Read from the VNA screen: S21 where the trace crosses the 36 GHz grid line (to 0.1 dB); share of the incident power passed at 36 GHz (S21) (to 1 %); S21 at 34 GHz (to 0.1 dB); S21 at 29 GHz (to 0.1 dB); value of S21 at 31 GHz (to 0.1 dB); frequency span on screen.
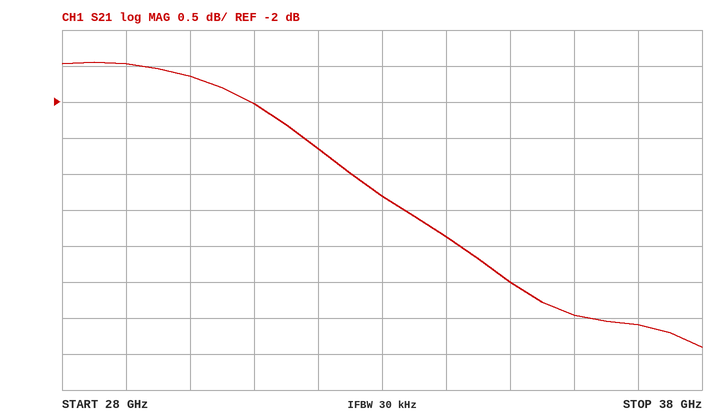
-5.0 dB
32 %
-3.9 dB
-1.5 dB
-2.0 dB
10 GHz
